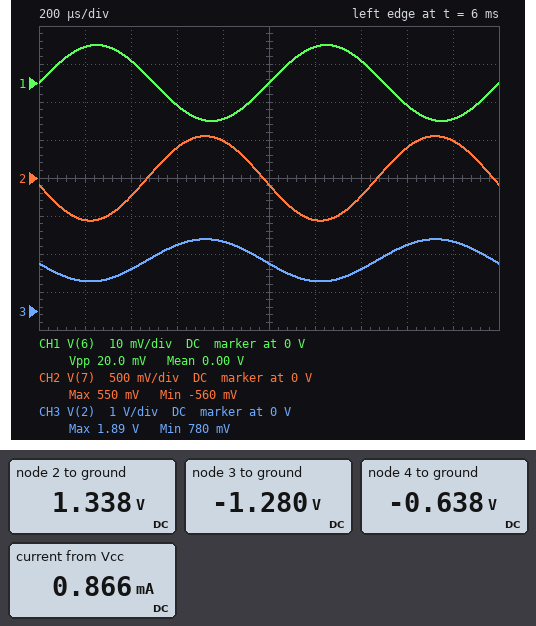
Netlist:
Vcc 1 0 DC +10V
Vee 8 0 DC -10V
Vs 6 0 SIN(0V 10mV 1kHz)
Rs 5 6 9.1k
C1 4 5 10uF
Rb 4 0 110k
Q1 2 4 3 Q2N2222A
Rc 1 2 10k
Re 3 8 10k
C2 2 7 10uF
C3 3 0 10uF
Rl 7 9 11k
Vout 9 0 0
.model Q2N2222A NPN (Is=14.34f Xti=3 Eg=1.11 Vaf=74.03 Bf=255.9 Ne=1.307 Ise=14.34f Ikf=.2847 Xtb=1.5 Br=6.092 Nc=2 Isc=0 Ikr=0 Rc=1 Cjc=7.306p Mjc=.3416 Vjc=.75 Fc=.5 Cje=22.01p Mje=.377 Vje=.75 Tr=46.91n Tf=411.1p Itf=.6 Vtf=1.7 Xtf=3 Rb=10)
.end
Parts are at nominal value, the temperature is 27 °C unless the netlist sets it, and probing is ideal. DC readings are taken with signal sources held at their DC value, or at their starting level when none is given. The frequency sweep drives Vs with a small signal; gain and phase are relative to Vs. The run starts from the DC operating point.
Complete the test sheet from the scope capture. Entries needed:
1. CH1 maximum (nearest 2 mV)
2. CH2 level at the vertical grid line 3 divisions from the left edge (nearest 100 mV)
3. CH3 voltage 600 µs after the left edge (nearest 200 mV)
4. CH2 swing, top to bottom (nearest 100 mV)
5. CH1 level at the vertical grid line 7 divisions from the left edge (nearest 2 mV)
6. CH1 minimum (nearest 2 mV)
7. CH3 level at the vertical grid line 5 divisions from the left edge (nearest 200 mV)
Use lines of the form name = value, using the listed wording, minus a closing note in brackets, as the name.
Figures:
CH1 maximum = 10 mV
CH2 level at the vertical grid line 3 divisions from the left edge = 400 mV
CH3 voltage 600 µs after the left edge = 1.8 V
CH2 swing, top to bottom = 1.1 V
CH1 level at the vertical grid line 7 divisions from the left edge = 6 mV
CH1 minimum = -10 mV
CH3 level at the vertical grid line 5 divisions from the left edge = 1.2 V
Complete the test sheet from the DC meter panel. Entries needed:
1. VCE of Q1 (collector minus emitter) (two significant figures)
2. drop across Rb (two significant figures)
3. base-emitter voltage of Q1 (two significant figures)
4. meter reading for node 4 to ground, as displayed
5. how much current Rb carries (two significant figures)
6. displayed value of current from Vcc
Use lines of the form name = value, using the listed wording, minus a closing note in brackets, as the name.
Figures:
VCE of Q1 (collector minus emitter) = 2.6 V
drop across Rb = 640 mV
base-emitter voltage of Q1 = 640 mV
meter reading for node 4 to ground, as displayed = -0.638 V
how much current Rb carries = 5.8 µA
displayed value of current from Vcc = 0.866 mA
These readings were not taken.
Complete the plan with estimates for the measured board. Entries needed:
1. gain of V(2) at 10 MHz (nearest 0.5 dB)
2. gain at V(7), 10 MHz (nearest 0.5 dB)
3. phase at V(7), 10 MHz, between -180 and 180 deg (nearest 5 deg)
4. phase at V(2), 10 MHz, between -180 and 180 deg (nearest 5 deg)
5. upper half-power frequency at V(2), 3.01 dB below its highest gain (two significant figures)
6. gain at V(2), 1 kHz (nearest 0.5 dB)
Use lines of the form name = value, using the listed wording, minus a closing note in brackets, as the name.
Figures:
gain of V(2) at 10 MHz = -9.5 dB
gain at V(7), 10 MHz = -9.5 dB
phase at V(7), 10 MHz, between -180 and 180 deg = 85 deg
phase at V(2), 10 MHz, between -180 and 180 deg = 85 deg
upper half-power frequency at V(2), 3.01 dB below its highest gain = 61 kHz
gain at V(2), 1 kHz = 35.0 dB
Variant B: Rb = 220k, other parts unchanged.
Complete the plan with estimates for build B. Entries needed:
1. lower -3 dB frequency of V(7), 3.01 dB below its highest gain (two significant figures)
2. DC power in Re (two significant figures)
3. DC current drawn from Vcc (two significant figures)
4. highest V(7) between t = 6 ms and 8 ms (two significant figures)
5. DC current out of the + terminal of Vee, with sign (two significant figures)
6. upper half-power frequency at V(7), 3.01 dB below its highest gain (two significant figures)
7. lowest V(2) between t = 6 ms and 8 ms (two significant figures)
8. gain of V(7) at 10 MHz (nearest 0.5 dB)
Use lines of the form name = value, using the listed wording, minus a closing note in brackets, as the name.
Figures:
lower -3 dB frequency of V(7), 3.01 dB below its highest gain = 180 Hz
DC power in Re = 6.7 mW
DC current drawn from Vcc = 810 µA
highest V(7) between t = 6 ms and 8 ms = 550 mV
DC current out of the + terminal of Vee, with sign = -820 µA
upper half-power frequency at V(7), 3.01 dB below its highest gain = 68 kHz
lowest V(2) between t = 6 ms and 8 ms = 1.3 V
gain of V(7) at 10 MHz = -8.5 dB
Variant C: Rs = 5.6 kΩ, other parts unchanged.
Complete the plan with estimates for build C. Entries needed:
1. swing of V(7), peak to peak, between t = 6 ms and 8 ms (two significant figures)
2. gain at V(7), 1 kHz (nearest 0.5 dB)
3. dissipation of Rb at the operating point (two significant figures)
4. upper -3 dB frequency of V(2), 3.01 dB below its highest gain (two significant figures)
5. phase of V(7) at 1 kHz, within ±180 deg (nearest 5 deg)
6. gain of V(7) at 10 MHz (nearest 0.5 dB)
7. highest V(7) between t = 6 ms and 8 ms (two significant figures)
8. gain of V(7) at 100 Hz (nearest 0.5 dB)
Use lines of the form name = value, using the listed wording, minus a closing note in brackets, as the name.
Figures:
swing of V(7), peak to peak, between t = 6 ms and 8 ms = 1.5 V
gain at V(7), 1 kHz = 37.5 dB
dissipation of Rb at the operating point = 3.7 µW
upper -3 dB frequency of V(2), 3.01 dB below its highest gain = 74 kHz
phase of V(7) at 1 kHz, within ±180 deg = -165 deg
gain of V(7) at 10 MHz = -5.0 dB
highest V(7) between t = 6 ms and 8 ms = 720 mV
gain of V(7) at 100 Hz = 29.0 dB
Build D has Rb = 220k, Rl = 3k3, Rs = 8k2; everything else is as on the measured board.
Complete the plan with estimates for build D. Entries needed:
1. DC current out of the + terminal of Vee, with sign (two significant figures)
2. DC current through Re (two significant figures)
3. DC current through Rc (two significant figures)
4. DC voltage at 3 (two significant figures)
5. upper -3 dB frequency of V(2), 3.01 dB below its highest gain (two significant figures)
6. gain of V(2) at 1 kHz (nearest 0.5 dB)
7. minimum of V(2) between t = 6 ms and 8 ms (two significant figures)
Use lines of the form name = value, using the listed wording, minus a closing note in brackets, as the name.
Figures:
DC current out of the + terminal of Vee, with sign = -820 µA
DC current through Re = 820 µA
DC current through Rc = 810 µA
DC voltage at 3 = -1.8 V
upper -3 dB frequency of V(2), 3.01 dB below its highest gain = 130 kHz
gain of V(2) at 1 kHz = 29.0 dB
minimum of V(2) between t = 6 ms and 8 ms = 1.6 V
